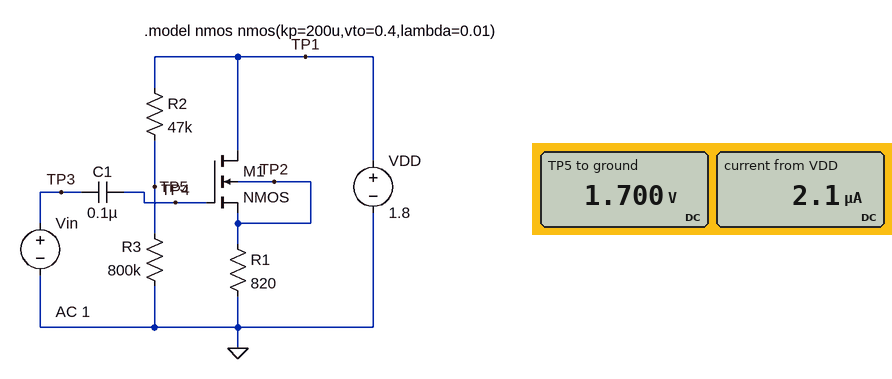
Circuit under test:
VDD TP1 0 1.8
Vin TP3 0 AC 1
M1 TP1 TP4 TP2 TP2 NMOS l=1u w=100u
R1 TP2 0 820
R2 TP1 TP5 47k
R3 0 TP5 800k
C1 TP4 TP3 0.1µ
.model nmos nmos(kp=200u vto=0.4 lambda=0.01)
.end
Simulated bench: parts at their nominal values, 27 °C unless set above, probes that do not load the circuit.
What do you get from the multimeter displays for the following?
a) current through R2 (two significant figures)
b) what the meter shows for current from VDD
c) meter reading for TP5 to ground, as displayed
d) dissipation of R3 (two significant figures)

2.1 µA
2.1 µA
1.700 V
3.6 µW
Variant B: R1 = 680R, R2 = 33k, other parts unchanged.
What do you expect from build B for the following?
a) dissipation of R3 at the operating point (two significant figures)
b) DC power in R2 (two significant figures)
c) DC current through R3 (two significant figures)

3.7 µW
150 nW
2.2 µA
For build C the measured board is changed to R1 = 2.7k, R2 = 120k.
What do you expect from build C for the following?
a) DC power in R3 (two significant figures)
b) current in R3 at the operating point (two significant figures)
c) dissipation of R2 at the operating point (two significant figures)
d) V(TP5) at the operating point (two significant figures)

3.1 µW
2.0 µA
460 nW
1.6 V
